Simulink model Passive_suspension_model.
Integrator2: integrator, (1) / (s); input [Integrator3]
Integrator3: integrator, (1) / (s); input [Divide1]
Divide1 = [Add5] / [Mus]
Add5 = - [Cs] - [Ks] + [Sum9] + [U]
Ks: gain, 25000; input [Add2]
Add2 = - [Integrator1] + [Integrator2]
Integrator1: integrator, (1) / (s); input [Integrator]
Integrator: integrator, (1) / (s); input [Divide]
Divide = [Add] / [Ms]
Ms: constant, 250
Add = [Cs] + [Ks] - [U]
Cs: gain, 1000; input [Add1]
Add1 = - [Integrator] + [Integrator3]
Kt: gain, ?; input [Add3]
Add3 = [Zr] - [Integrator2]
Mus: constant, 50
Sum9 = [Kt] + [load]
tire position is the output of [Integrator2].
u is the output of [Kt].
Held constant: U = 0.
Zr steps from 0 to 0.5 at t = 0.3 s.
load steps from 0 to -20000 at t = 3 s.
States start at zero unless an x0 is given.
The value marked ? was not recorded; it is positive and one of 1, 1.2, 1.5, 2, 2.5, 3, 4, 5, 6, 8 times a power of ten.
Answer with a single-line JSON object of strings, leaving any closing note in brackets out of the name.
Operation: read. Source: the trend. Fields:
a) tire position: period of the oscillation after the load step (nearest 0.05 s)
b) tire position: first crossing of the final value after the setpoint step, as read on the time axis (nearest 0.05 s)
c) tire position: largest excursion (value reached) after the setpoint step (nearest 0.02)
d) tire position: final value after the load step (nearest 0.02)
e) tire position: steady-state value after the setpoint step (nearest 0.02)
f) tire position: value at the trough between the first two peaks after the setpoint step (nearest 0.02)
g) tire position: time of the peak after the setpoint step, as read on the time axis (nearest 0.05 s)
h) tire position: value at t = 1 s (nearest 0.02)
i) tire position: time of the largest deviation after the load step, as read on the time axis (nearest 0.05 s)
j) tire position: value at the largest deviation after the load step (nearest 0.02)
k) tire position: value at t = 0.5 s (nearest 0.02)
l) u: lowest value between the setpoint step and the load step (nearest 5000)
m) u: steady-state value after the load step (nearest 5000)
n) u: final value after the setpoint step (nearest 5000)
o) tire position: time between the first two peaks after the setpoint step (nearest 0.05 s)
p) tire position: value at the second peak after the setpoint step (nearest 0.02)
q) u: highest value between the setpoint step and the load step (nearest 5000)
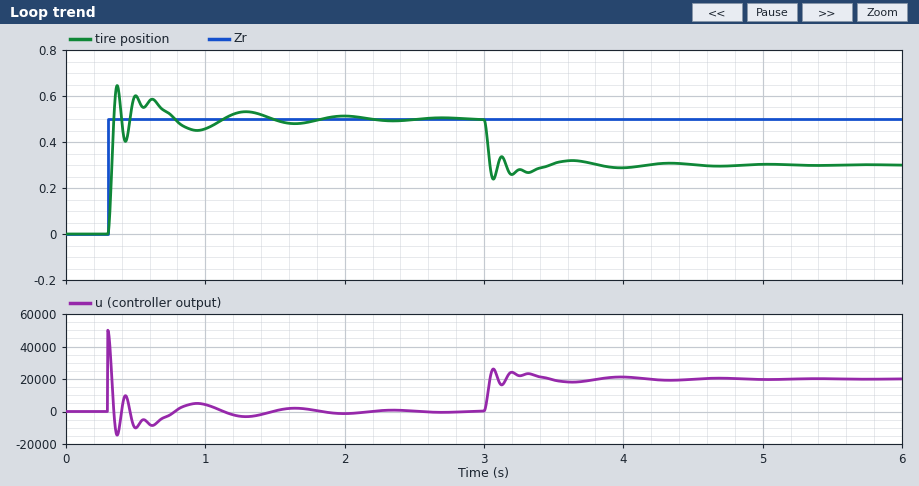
{"tire position: period of the oscillation after the load step": "0.15 s", "tire position: first crossing of the final value after the setpoint step, as read on the time axis": "0.35 s", "tire position: largest excursion (value reached) after the setpoint step": "0.64", "tire position: final value after the load step": "0.30", "tire position: steady-state value after the setpoint step": "0.50", "tire position: value at the trough between the first two peaks after the setpoint step": "0.40", "tire position: time of the peak after the setpoint step, as read on the time axis": "0.35 s", "tire position: value at t = 1 s": "0.46", "tire position: time of the largest deviation after the load step, as read on the time axis": "3.05 s", "tire position: value at the largest deviation after the load step": "0.24", "tire position: value at t = 0.5 s": "0.60", "u: lowest value between the setpoint step and the load step": "-15000", "u: steady-state value after the load step": "20000", "u: final value after the setpoint step": "0", "tire position: time between the first two peaks after the setpoint step": "0.15 s", "tire position: value at the second peak after the setpoint step": "0.60", "u: highest value between the setpoint step and the load step": "50000"}
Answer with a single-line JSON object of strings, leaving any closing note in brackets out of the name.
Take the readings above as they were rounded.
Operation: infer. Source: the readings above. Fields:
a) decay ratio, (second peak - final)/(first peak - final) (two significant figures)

{"decay ratio, (second peak - final)/(first peak - final)": "0.71"}
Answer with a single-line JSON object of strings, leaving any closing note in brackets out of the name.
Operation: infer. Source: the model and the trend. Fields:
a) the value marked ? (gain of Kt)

{"the value marked ?": "100000"}
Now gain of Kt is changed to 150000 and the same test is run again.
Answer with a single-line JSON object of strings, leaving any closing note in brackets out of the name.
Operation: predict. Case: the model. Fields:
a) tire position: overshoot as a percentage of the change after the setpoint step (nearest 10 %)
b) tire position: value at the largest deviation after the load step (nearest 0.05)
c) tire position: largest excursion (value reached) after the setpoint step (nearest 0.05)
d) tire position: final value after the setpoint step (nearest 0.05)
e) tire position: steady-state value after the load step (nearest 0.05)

{"tire position: overshoot as a percentage of the change after the setpoint step": "40 %", "tire position: value at the largest deviation after the load step": "0.30", "tire position: largest excursion (value reached) after the setpoint step": "0.70", "tire position: final value after the setpoint step": "0.50", "tire position: steady-state value after the load step": "0.35"}
